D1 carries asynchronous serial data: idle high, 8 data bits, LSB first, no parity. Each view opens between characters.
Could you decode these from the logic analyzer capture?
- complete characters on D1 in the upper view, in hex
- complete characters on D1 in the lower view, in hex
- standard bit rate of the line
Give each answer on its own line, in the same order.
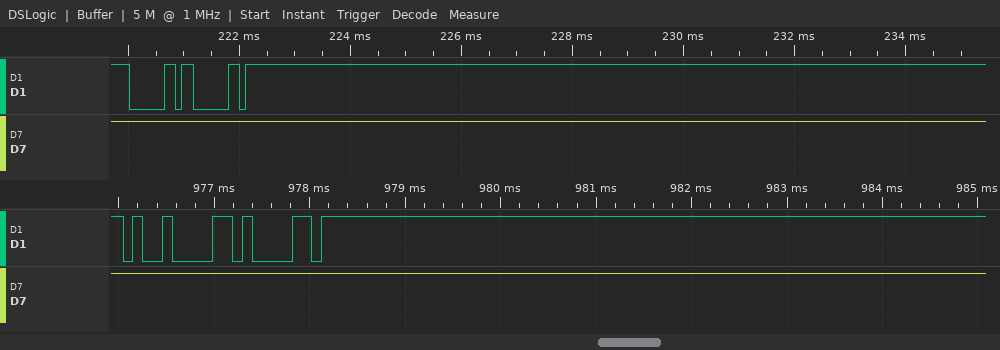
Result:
60, 60
09, 61
9600 baud
